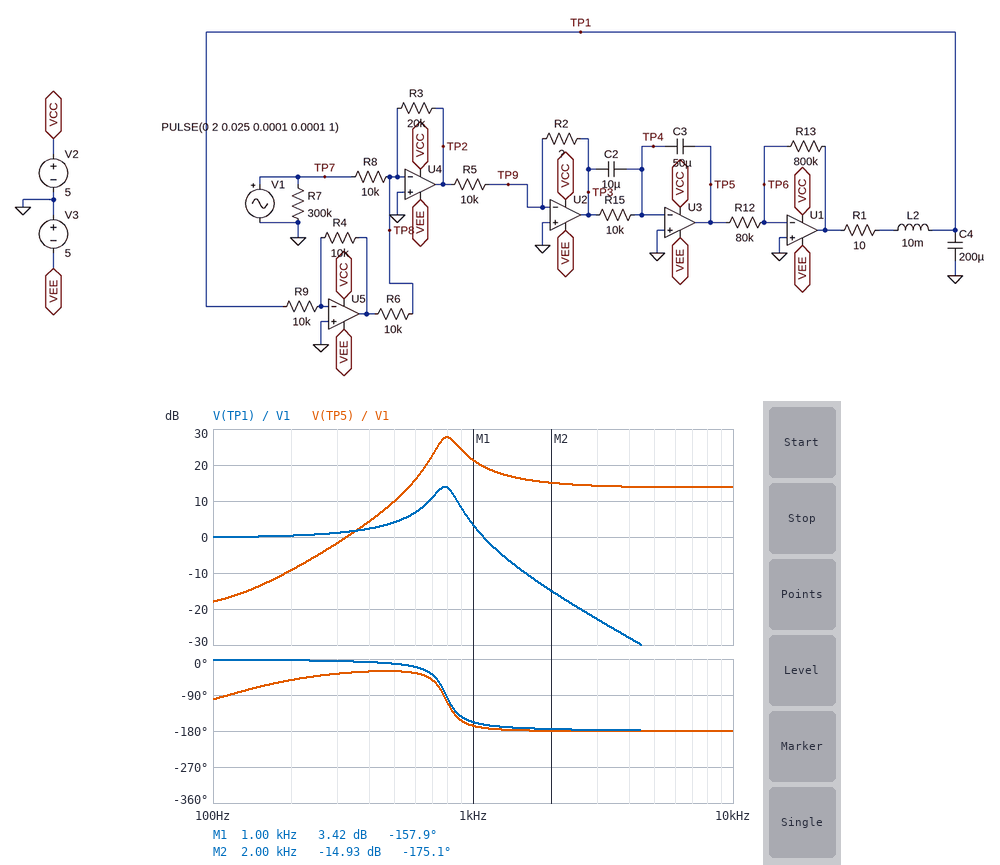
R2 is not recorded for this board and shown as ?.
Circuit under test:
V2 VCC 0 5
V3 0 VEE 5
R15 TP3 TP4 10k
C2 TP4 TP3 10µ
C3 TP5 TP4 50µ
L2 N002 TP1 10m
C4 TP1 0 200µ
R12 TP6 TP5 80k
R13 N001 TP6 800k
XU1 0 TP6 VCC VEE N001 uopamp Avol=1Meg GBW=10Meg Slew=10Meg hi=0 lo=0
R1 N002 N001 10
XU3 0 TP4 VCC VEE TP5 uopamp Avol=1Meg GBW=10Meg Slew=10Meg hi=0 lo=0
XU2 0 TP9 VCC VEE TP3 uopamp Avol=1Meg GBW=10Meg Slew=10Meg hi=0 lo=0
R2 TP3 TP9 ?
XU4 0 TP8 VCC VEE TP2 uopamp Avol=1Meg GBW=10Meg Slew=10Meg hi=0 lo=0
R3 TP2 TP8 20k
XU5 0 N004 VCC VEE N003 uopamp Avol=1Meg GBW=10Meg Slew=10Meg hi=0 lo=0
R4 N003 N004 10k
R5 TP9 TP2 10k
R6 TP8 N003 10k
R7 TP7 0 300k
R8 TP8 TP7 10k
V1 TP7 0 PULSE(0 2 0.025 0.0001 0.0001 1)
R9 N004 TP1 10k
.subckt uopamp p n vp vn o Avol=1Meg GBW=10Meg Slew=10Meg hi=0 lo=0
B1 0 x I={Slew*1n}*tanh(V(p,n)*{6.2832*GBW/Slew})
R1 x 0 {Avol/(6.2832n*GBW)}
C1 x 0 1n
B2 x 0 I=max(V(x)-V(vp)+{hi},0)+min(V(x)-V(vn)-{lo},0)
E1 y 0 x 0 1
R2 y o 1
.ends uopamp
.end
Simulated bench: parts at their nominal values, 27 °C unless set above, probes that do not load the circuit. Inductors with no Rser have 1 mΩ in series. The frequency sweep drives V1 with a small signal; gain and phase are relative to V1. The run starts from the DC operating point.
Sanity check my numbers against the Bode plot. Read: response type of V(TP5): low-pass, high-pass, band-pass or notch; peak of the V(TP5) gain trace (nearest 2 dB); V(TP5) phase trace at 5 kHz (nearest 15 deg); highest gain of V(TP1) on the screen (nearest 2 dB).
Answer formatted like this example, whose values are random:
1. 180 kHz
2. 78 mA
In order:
1. high-pass
2. 28 dB
3. -180 deg
4. 14 dB
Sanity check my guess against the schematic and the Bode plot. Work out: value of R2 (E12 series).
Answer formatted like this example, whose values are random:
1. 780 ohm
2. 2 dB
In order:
1. 120 kΩ
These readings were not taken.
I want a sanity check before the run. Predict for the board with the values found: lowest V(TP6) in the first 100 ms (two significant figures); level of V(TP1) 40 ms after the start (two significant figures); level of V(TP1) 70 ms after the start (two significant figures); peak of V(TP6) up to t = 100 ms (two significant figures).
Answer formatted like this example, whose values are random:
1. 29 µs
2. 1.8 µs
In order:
1. -500 mV
2. 2.0 V
3. 2.0 V
4. 450 mV
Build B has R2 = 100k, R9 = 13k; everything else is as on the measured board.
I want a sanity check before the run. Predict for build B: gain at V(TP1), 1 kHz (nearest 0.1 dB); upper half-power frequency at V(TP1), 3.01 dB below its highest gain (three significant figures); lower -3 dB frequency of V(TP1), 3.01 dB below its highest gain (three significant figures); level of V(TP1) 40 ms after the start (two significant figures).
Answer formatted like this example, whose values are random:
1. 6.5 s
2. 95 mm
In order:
1. -1.7 dB
2. 699 Hz
3. 540 Hz
4. 2.5 V
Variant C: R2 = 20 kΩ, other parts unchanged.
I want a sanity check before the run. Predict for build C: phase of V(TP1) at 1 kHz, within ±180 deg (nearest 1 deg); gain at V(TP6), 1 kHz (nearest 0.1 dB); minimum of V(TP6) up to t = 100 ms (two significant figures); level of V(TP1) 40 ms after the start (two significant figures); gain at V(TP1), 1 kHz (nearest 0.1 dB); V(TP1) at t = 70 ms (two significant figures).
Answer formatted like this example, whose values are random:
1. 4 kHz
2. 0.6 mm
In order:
1. -170 deg
2. -61.0 dB
3. -490 mV
4. 1.8 V
5. -19.0 dB
6. 1.9 V
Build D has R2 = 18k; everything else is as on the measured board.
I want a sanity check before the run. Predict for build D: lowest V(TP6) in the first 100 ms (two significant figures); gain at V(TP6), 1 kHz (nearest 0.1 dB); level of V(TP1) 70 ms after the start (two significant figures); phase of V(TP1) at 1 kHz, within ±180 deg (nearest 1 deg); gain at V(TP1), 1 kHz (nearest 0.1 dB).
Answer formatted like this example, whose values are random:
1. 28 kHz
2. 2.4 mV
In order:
1. -480 mV
2. -62.0 dB
3. 1.8 V
4. -170 deg
5. -20.0 dB
